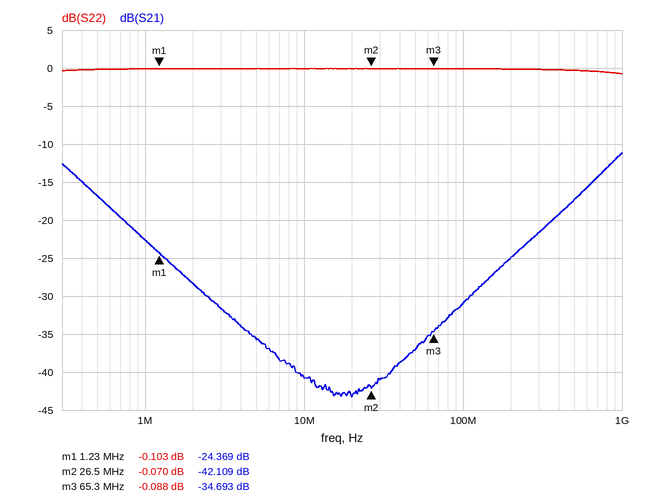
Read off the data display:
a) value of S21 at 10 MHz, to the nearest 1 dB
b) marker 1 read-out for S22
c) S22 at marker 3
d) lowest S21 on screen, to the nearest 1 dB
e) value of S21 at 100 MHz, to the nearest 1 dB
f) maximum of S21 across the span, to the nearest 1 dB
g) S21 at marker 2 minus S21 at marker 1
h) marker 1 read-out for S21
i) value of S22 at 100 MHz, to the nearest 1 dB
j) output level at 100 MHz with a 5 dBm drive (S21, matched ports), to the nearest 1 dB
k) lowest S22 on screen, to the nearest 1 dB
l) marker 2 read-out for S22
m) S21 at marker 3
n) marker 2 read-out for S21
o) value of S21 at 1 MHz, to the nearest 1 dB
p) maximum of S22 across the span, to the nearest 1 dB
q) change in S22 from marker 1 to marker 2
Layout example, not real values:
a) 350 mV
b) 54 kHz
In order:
a) -41 dB
b) -0.103 dB
c) -0.088 dB
d) -43 dB
e) -31 dB
f) -11 dB
g) -17.740 dB
h) -24.369 dB
i) 0 dB
j) -26 dBm
k) -1 dB
l) -0.070 dB
m) -34.693 dB
n) -42.109 dB
o) -23 dB
p) 0 dB
q) 0.033 dB
